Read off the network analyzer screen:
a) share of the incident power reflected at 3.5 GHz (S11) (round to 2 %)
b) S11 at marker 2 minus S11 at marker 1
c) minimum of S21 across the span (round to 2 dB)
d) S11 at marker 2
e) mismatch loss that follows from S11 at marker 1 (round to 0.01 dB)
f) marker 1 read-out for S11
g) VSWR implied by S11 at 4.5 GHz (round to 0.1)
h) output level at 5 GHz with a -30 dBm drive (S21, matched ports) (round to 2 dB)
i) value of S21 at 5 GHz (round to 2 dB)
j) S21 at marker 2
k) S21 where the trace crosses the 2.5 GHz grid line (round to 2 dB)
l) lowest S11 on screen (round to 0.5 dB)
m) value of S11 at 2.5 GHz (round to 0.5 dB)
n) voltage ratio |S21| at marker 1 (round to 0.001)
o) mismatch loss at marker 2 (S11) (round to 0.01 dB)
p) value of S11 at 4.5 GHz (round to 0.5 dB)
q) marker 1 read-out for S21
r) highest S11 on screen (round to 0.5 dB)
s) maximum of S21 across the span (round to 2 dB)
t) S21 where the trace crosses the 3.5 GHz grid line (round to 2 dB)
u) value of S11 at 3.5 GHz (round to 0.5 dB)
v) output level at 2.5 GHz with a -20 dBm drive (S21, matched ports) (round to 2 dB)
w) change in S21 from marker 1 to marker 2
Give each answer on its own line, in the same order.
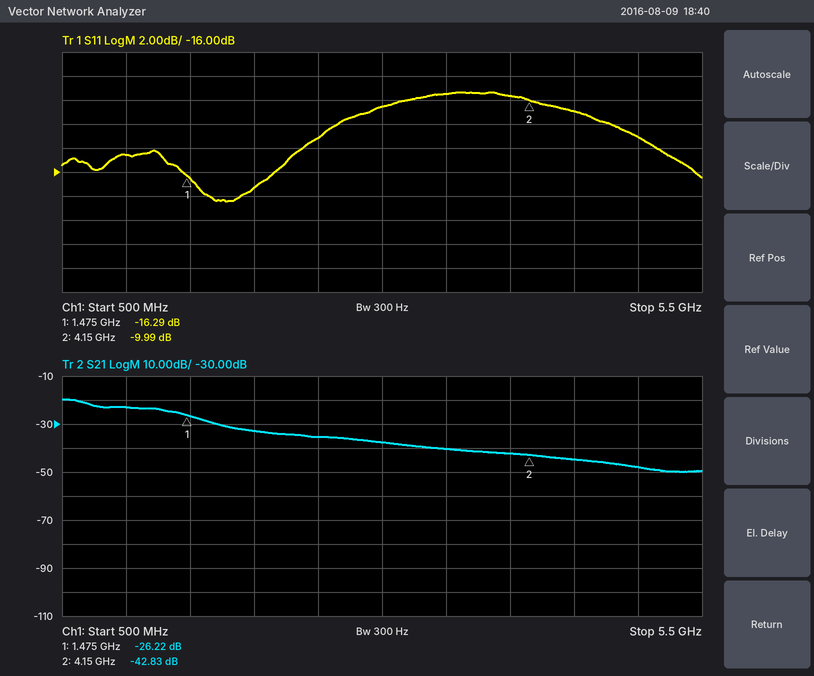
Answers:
12 %
6.30 dB
-50 dB
-9.99 dB
0.10 dB
-16.29 dB
1.8
-78 dBm
-48 dB
-42.83 dB
-36 dB
-18.5 dB
-13.0 dB
0.049
0.46 dB
-11.0 dB
-26.22 dB
-9.5 dB
-20 dB
-40 dB
-9.5 dB
-56 dBm
-16.61 dB
